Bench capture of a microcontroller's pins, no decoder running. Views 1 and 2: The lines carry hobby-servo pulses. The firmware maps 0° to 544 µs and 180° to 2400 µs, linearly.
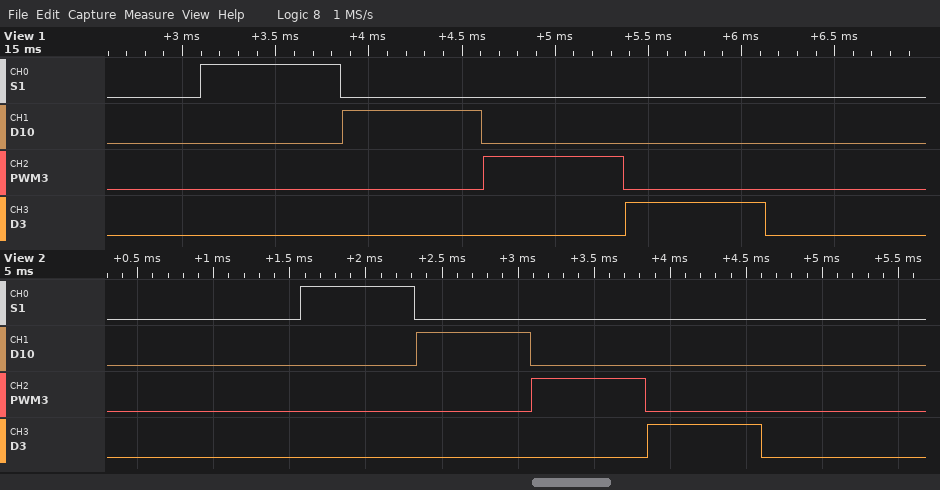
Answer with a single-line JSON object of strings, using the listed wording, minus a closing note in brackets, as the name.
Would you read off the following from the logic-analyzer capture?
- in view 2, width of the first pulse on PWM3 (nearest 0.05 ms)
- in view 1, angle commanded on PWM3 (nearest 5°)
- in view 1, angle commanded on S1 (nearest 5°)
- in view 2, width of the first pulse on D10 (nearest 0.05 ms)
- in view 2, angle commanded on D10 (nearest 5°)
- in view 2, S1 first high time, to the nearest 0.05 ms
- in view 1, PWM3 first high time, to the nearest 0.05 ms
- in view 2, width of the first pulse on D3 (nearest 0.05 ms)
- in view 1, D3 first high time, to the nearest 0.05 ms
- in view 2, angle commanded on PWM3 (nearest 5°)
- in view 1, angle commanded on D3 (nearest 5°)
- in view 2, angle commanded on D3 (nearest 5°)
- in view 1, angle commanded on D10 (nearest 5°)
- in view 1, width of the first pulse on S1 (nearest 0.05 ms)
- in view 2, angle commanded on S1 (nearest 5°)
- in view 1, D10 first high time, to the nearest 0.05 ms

{"in view 2, width of the first pulse on PWM3": "0.75 ms", "in view 1, angle commanded on PWM3": "20°", "in view 1, angle commanded on S1": "20°", "in view 2, width of the first pulse on D10": "0.75 ms", "in view 2, angle commanded on D10": "20°", "in view 2, S1 first high time, to the nearest 0.05 ms": "0.75 ms", "in view 1, PWM3 first high time, to the nearest 0.05 ms": "0.75 ms", "in view 2, width of the first pulse on D3": "0.75 ms", "in view 1, D3 first high time, to the nearest 0.05 ms": "0.75 ms", "in view 2, angle commanded on PWM3": "20°", "in view 1, angle commanded on D3": "20°", "in view 2, angle commanded on D3": "20°", "in view 1, angle commanded on D10": "20°", "in view 1, width of the first pulse on S1": "0.75 ms", "in view 2, angle commanded on S1": "20°", "in view 1, D10 first high time, to the nearest 0.05 ms": "0.75 ms"}
